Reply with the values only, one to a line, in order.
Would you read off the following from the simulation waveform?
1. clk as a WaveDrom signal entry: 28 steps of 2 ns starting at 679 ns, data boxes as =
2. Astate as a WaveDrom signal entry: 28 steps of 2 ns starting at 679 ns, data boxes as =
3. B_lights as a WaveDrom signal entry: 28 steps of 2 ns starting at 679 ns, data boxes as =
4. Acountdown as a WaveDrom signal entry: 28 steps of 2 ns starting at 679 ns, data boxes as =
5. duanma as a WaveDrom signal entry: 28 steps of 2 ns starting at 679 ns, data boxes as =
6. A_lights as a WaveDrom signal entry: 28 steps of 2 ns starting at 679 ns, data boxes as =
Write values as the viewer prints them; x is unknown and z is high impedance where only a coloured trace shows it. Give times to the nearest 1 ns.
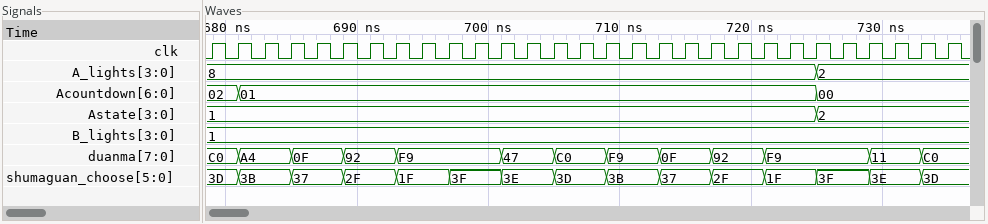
{name: 'clk', wave: 'p...........................'}
{name: 'Astate', wave: '=......................=....', data: '1 2'}
{name: 'B_lights', wave: '=...........................', data: '1'}
{name: 'Acountdown', wave: '==.....................=....', data: '02 01 00'}
{name: 'duanma', wave: '==.=.=.=...=.=.=.=.=.=...=.=', data: 'C0 A4 0F 92 F9 47 C0 F9 0F 92 F9 11 C0'}
{name: 'A_lights', wave: '=......................=....', data: '8 2'}
